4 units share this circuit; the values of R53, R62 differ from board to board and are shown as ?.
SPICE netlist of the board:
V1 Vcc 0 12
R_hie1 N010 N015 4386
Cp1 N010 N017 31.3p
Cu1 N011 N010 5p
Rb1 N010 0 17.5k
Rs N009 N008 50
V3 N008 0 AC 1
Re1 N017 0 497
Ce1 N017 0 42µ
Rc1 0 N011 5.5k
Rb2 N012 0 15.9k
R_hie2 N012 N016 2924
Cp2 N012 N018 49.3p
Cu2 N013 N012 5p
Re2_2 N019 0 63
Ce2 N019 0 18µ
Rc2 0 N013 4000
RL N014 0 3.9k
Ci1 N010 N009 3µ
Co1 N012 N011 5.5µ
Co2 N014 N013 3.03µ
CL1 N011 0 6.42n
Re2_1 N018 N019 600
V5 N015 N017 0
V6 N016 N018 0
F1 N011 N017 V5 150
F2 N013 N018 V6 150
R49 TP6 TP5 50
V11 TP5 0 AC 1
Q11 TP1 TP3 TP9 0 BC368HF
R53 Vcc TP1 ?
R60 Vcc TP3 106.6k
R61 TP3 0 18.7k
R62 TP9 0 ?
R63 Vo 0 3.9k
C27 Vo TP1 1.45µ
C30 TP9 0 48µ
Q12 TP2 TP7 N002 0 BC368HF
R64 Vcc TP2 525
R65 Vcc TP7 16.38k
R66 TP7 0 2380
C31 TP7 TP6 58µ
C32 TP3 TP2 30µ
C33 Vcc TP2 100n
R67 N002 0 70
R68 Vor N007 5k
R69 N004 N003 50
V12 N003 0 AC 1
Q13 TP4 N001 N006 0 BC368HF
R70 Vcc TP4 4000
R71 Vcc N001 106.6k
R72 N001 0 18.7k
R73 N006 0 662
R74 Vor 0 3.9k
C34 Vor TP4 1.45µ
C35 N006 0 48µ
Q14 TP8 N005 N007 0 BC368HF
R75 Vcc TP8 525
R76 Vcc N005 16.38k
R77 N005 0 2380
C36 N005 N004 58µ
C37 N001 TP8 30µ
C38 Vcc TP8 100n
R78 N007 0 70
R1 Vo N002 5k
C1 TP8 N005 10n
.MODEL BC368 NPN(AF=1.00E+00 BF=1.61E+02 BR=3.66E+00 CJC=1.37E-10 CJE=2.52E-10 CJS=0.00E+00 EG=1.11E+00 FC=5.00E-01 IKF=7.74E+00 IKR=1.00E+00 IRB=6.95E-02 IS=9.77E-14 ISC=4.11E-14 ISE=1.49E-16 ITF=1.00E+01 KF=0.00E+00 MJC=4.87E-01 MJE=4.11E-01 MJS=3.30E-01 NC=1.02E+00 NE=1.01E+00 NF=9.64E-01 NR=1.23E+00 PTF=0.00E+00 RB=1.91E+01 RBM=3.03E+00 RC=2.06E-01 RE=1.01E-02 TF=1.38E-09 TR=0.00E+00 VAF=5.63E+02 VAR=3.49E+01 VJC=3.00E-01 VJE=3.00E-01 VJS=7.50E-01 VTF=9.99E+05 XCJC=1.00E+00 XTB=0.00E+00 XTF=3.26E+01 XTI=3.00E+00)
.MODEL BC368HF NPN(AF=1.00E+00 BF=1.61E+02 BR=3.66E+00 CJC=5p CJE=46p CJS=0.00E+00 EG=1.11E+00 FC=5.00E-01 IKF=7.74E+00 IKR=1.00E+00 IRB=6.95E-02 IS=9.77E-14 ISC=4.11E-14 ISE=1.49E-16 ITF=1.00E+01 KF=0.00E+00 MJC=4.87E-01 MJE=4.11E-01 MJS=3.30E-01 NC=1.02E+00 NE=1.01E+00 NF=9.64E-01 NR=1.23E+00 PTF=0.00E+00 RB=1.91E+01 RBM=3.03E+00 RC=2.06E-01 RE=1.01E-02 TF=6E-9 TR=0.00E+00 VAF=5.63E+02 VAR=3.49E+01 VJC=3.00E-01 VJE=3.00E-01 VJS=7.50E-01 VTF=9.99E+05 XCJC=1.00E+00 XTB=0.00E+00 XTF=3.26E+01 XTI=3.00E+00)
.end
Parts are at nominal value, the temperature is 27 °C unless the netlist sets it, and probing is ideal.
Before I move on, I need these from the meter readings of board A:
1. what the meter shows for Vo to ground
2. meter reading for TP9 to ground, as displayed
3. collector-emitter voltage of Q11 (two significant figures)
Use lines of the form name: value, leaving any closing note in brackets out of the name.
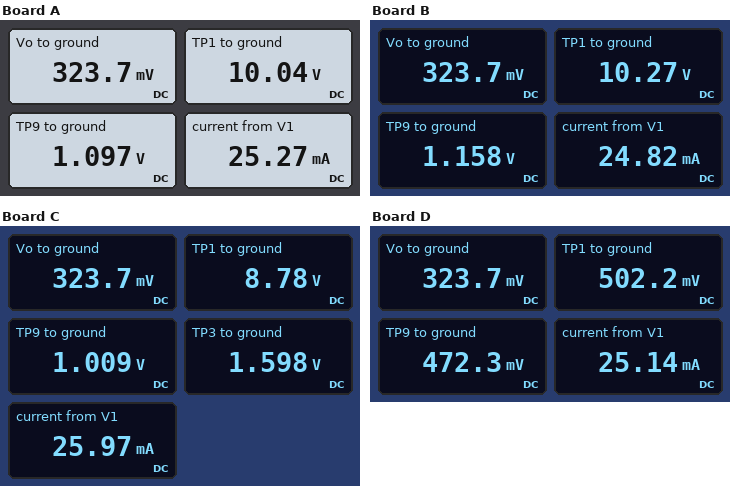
what the meter shows for Vo to ground: 323.7 mV
meter reading for TP9 to ground, as displayed: 1.097 V
collector-emitter voltage of Q11: 8.9 V
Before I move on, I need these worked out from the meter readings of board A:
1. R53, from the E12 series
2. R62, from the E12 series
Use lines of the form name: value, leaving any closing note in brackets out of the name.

R53, from the E12 series: 1.8 kΩ
R62, from the E12 series: 1 kΩ
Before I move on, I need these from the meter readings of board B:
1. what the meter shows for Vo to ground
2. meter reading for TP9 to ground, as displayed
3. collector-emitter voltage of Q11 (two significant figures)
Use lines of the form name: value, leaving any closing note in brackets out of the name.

what the meter shows for Vo to ground: 323.7 mV
meter reading for TP9 to ground, as displayed: 1.158 V
collector-emitter voltage of Q11: 9.1 V
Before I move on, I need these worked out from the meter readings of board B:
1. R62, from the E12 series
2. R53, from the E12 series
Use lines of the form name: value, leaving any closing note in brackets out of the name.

R62, from the E12 series: 1.8 kΩ
R53, from the E12 series: 2.7 kΩ
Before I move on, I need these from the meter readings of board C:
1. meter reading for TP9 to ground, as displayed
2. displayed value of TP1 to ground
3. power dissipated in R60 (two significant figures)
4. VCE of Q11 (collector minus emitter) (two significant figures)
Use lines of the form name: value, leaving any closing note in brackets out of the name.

meter reading for TP9 to ground, as displayed: 1.009 V
displayed value of TP1 to ground: 8.78 V
power dissipated in R60: 1.0 mW
VCE of Q11 (collector minus emitter): 7.8 V
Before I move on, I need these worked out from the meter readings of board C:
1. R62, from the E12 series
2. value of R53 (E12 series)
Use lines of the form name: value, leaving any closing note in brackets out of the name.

R62, from the E12 series: 560 Ω
value of R53: 1.8 kΩ
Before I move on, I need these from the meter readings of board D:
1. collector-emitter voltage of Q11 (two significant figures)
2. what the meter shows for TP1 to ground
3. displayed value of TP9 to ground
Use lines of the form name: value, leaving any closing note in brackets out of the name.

collector-emitter voltage of Q11: 30 mV
what the meter shows for TP1 to ground: 502.2 mV
displayed value of TP9 to ground: 472.3 mV
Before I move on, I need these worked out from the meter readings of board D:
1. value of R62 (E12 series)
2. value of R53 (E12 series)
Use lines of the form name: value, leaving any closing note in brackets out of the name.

value of R62: 470 Ω
value of R53: 12 kΩ
